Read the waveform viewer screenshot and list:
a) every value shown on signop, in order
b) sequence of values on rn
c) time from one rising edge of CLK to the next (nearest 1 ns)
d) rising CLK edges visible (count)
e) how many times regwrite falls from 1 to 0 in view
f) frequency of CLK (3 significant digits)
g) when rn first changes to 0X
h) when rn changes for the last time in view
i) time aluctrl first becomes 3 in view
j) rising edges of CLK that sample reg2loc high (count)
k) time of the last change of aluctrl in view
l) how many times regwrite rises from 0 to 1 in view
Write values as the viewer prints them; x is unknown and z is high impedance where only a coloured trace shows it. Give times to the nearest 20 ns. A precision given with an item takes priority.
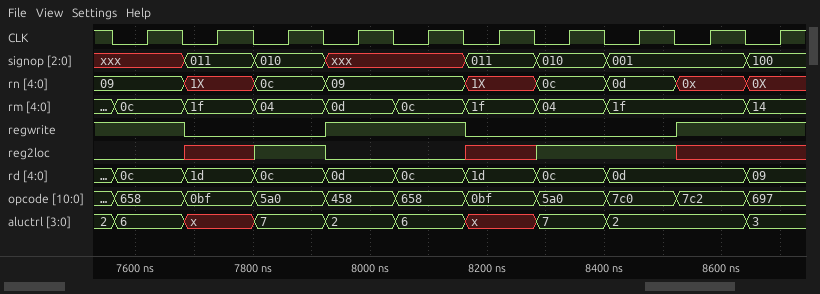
xxx, 011, 010, xxx, 011, 010, 001, 100
09, 1X, 0c, 09, 1X, 0c, 0d, 0x, 0X
120 ns
10
2
8.33 MHz
8640 ns
8640 ns
8640 ns
3
8640 ns
2
